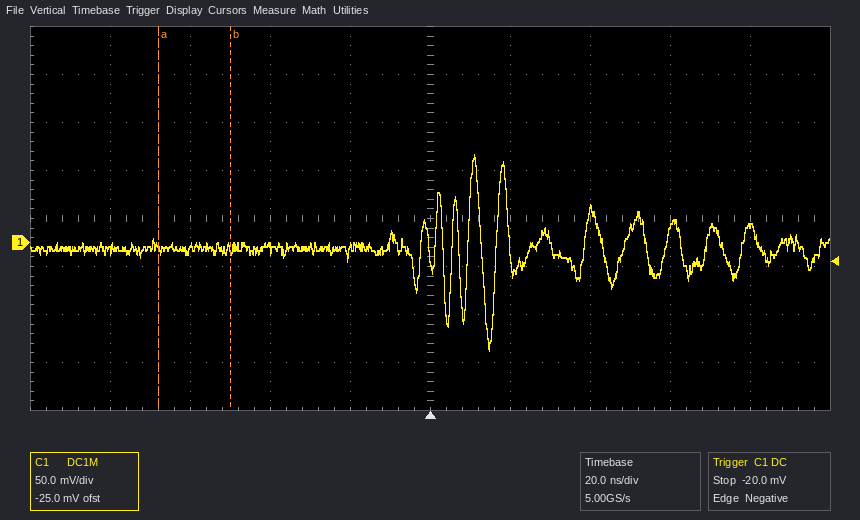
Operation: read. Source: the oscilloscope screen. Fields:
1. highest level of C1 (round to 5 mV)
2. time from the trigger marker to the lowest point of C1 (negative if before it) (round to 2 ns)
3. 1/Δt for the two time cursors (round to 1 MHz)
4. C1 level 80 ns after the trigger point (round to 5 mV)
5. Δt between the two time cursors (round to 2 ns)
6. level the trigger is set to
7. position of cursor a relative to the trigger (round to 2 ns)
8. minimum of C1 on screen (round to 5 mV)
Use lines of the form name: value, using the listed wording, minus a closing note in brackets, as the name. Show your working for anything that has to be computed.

highest level of C1: 90 mV
time from the trigger marker to the lowest point of C1 (negative if before it): +14 ns
1/Δt for the two time cursors: 1 / 18 ns ≈ 56 MHz
C1 level 80 ns after the trigger point: 15 mV
Δt between the two time cursors: 18 ns
level the trigger is set to: -20.0 mV
position of cursor a relative to the trigger: -68 ns
minimum of C1 on screen: -110 mV
